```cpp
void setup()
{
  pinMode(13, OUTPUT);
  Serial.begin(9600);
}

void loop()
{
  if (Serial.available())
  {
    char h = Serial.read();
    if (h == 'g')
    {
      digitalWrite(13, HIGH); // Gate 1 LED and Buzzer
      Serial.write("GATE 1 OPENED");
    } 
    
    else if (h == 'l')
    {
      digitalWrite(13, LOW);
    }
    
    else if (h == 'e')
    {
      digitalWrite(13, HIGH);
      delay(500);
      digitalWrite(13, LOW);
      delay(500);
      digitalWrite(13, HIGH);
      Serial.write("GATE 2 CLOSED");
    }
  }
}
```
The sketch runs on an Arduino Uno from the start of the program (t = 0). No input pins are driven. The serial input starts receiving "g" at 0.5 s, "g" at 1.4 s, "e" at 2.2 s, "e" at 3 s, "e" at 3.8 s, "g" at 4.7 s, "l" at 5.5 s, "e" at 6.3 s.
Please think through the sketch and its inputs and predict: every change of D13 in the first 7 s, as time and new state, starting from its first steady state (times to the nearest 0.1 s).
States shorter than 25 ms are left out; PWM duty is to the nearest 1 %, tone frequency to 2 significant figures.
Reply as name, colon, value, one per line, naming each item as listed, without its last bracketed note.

every change of D13 in the first 7 s, as time and new state, starting from its first steady state: 0 s low; 0.5 s high; 2.7 s low; 3.2 s high; 3.7 s low; 4.2 s high; 4.7 s low; 5.2 s high; 5.5 s low; 6.3 s high; 6.8 s low
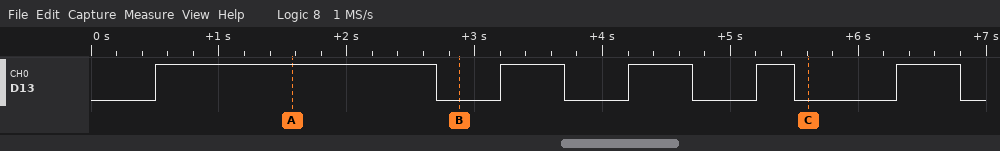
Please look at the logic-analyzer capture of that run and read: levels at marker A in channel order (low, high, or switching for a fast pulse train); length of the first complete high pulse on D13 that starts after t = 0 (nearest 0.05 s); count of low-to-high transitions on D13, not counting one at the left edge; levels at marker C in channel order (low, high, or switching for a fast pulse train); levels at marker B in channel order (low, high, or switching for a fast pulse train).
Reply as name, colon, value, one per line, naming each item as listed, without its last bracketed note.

levels at marker A in channel order: D13 high
length of the first complete high pulse on D13 that starts after t = 0: 2.20 s
count of low-to-high transitions on D13, not counting one at the left edge: 5
levels at marker C in channel order: D13 low
levels at marker B in channel order: D13 low
